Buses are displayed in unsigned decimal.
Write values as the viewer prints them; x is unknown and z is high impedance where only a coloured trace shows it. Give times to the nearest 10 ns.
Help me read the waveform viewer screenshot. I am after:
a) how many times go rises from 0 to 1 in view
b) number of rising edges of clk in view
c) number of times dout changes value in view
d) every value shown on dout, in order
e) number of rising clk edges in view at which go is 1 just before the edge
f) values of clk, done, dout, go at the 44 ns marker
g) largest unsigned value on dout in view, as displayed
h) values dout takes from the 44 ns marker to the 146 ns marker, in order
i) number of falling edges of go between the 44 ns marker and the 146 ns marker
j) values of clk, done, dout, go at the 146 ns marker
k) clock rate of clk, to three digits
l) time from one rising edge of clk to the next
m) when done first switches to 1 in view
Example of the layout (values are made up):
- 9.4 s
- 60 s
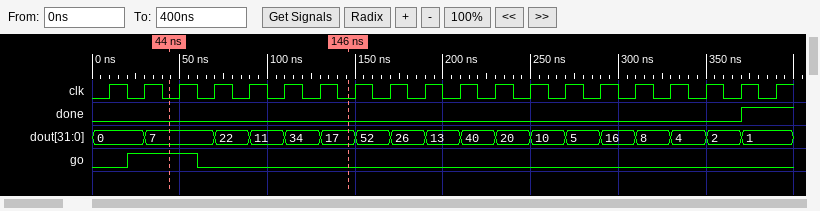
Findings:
- 1
- 20
- 17
- 0, 7, 22, 11, 34, 17, 52, 26, 13, 40, 20, 10, 5, 16, 8, 4, 2, 1
- 2
- clk=0, done=0, dout=7, go=1
- 52
- 7, 22, 11, 34, 17
- 1
- clk=0, done=0, dout=17, go=0
- 50.0 MHz
- 20 ns
- 370 ns
